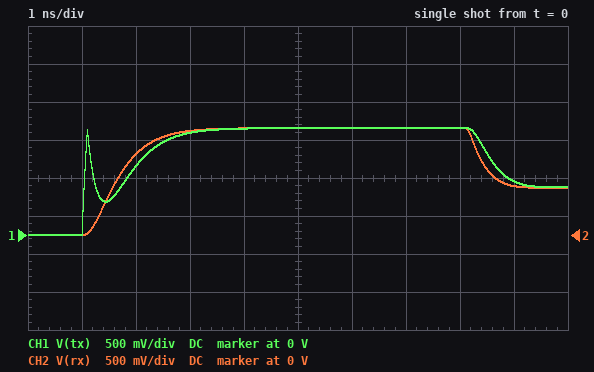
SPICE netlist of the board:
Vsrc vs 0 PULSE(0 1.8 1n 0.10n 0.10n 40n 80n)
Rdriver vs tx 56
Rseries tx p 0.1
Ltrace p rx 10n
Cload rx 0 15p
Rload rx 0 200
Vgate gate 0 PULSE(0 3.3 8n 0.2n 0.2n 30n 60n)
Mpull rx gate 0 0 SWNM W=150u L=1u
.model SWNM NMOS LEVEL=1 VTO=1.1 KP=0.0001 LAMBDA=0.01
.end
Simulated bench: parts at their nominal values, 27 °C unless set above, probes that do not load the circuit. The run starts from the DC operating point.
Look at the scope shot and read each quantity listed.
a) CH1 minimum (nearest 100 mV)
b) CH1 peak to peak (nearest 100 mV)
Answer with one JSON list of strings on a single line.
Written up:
["0 V", "1.4 V"]
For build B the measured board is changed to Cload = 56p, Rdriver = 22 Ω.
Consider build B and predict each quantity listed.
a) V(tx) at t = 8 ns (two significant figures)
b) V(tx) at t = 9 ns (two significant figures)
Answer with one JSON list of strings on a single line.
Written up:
["1.6 V", "1.4 V"]
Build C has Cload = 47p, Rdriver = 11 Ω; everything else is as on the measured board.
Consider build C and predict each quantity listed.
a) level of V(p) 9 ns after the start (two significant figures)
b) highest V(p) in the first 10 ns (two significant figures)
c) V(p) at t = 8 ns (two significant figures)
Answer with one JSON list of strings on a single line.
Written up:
["1.5 V", "1.9 V", "1.7 V"]
